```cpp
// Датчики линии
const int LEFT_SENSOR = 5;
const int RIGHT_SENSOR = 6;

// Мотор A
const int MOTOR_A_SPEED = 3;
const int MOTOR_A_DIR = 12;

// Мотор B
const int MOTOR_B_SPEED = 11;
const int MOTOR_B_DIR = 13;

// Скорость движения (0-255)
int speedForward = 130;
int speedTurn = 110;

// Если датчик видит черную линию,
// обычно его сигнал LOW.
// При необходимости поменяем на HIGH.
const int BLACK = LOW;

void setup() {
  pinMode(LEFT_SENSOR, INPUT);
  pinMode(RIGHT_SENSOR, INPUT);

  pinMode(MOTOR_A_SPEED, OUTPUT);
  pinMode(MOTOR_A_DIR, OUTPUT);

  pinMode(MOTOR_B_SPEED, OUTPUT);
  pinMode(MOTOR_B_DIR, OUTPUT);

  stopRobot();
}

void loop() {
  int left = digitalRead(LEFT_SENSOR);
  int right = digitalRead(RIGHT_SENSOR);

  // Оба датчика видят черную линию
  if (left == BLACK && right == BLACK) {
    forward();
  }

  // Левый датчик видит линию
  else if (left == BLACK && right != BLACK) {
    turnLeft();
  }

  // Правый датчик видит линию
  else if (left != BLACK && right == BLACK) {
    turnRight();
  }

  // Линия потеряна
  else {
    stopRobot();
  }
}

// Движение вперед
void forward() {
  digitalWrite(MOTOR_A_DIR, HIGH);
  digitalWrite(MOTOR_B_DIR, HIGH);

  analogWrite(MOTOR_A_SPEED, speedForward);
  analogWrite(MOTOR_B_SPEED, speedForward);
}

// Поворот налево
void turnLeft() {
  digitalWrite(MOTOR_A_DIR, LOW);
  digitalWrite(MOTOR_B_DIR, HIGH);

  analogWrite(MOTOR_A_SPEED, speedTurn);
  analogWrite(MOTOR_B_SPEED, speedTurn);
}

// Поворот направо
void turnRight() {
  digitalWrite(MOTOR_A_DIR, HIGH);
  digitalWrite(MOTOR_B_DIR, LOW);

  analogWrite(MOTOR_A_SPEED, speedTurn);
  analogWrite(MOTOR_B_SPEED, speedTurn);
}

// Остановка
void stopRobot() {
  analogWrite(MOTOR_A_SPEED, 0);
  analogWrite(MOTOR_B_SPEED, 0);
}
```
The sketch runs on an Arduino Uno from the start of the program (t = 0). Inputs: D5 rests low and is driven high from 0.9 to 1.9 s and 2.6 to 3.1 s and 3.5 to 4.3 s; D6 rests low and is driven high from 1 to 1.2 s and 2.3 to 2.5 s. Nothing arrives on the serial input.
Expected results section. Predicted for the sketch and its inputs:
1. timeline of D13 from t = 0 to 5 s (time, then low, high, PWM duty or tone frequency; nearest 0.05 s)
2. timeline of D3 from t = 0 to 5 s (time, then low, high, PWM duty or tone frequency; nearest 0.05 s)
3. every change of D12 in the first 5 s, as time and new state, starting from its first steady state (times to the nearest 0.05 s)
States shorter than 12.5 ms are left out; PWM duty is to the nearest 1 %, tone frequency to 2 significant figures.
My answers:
0 s high; 0.9 s low; 1.9 s high; 2.6 s low; 3.1 s high; 3.5 s low; 4.3 s high
0 s PWM 51 %; 0.9 s PWM 43 %; 1 s low; 1.2 s PWM 43 %; 1.9 s PWM 51 %; 2.3 s PWM 43 %; 2.5 s PWM 51 %; 2.6 s PWM 43 %; 3.1 s PWM 51 %; 3.5 s PWM 43 %; 4.3 s PWM 51 %
0 s high; 2.3 s low; 2.5 s high
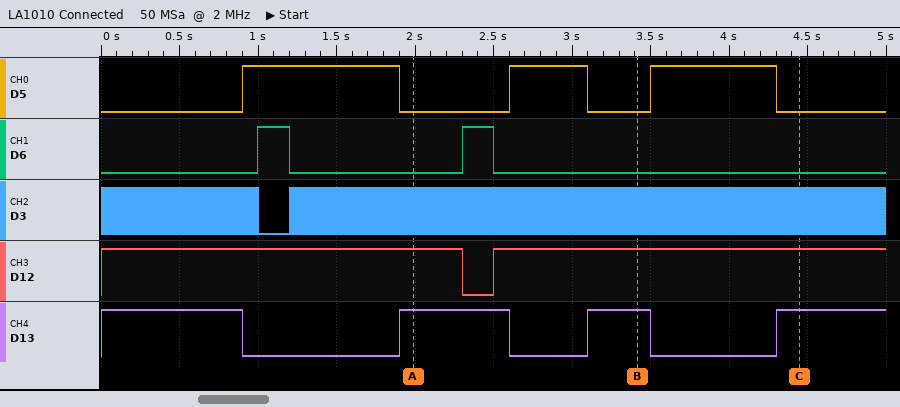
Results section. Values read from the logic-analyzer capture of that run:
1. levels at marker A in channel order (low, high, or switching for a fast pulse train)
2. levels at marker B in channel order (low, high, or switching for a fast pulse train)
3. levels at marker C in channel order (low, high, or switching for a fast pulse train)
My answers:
D5 low, D6 low, D3 switching, D12 high, D13 high
D5 low, D6 low, D3 switching, D12 high, D13 high
D5 low, D6 low, D3 switching, D12 high, D13 high
